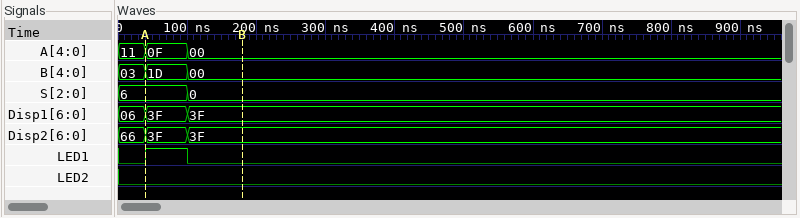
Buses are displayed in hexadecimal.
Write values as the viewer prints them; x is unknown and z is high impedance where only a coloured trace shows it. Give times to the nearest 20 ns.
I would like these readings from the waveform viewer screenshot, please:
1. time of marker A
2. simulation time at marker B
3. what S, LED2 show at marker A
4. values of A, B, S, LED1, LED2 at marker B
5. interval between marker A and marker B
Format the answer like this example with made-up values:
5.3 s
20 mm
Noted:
40 ns
180 ns
S=6, LED2=0
A=00, B=00, S=0, LED1=0, LED2=0
140 ns
